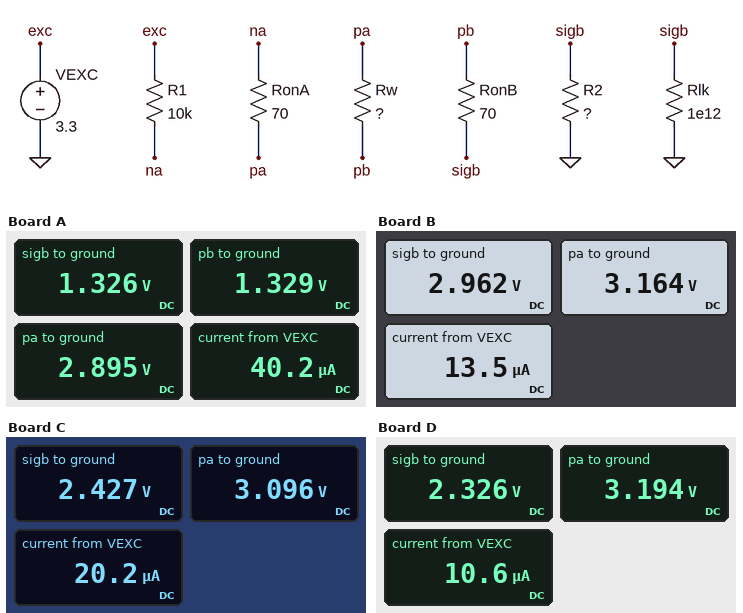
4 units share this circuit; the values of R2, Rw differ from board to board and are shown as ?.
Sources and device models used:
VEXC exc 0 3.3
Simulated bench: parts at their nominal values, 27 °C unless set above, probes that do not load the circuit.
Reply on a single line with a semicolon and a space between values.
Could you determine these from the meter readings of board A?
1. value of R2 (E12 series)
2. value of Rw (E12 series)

33 kΩ; 39 kΩ
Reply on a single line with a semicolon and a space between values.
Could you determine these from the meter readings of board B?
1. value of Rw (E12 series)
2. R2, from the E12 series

15 kΩ; 220 kΩ
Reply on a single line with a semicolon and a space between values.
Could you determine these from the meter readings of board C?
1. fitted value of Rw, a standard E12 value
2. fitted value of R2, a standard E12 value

33 kΩ; 120 kΩ
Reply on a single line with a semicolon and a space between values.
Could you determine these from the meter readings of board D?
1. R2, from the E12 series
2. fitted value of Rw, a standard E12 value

220 kΩ; 82 kΩ
